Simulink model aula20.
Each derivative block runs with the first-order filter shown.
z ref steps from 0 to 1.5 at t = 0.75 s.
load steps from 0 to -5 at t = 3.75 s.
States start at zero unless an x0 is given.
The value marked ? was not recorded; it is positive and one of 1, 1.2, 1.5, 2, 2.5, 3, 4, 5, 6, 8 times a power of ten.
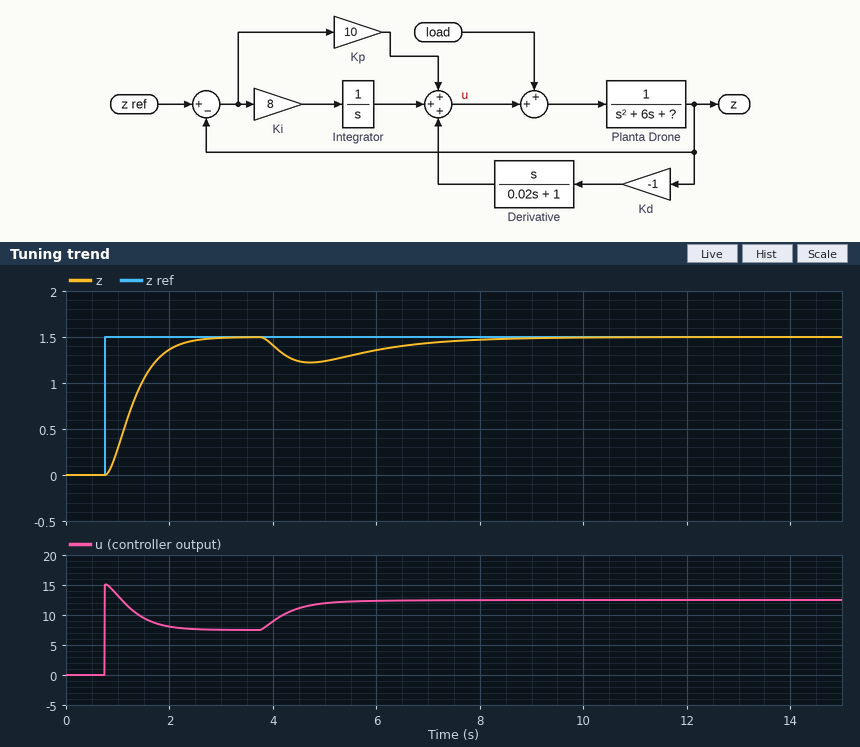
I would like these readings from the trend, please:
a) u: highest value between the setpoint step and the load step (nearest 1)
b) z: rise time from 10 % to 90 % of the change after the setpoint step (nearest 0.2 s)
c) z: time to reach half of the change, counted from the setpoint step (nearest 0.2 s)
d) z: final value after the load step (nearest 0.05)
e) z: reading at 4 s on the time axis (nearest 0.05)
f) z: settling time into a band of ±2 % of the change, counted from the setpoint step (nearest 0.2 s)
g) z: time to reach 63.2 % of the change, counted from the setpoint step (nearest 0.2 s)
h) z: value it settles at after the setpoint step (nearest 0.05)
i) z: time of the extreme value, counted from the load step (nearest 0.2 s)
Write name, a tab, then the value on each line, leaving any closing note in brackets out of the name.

u: highest value between the setpoint step and the load step	15
z: rise time from 10 % to 90 % of the change after the setpoint step	1.0 s
z: time to reach half of the change, counted from the setpoint step	0.6 s
z: final value after the load step	1.50
z: reading at 4 s on the time axis	1.40
z: settling time into a band of ±2 % of the change, counted from the setpoint step	1.8 s
z: time to reach 63.2 % of the change, counted from the setpoint step	0.6 s
z: value it settles at after the setpoint step	1.50
z: time of the extreme value, counted from the load step	1.0 s
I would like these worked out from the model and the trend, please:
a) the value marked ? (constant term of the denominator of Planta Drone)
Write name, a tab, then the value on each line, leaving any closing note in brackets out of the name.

the value marked ?	5
